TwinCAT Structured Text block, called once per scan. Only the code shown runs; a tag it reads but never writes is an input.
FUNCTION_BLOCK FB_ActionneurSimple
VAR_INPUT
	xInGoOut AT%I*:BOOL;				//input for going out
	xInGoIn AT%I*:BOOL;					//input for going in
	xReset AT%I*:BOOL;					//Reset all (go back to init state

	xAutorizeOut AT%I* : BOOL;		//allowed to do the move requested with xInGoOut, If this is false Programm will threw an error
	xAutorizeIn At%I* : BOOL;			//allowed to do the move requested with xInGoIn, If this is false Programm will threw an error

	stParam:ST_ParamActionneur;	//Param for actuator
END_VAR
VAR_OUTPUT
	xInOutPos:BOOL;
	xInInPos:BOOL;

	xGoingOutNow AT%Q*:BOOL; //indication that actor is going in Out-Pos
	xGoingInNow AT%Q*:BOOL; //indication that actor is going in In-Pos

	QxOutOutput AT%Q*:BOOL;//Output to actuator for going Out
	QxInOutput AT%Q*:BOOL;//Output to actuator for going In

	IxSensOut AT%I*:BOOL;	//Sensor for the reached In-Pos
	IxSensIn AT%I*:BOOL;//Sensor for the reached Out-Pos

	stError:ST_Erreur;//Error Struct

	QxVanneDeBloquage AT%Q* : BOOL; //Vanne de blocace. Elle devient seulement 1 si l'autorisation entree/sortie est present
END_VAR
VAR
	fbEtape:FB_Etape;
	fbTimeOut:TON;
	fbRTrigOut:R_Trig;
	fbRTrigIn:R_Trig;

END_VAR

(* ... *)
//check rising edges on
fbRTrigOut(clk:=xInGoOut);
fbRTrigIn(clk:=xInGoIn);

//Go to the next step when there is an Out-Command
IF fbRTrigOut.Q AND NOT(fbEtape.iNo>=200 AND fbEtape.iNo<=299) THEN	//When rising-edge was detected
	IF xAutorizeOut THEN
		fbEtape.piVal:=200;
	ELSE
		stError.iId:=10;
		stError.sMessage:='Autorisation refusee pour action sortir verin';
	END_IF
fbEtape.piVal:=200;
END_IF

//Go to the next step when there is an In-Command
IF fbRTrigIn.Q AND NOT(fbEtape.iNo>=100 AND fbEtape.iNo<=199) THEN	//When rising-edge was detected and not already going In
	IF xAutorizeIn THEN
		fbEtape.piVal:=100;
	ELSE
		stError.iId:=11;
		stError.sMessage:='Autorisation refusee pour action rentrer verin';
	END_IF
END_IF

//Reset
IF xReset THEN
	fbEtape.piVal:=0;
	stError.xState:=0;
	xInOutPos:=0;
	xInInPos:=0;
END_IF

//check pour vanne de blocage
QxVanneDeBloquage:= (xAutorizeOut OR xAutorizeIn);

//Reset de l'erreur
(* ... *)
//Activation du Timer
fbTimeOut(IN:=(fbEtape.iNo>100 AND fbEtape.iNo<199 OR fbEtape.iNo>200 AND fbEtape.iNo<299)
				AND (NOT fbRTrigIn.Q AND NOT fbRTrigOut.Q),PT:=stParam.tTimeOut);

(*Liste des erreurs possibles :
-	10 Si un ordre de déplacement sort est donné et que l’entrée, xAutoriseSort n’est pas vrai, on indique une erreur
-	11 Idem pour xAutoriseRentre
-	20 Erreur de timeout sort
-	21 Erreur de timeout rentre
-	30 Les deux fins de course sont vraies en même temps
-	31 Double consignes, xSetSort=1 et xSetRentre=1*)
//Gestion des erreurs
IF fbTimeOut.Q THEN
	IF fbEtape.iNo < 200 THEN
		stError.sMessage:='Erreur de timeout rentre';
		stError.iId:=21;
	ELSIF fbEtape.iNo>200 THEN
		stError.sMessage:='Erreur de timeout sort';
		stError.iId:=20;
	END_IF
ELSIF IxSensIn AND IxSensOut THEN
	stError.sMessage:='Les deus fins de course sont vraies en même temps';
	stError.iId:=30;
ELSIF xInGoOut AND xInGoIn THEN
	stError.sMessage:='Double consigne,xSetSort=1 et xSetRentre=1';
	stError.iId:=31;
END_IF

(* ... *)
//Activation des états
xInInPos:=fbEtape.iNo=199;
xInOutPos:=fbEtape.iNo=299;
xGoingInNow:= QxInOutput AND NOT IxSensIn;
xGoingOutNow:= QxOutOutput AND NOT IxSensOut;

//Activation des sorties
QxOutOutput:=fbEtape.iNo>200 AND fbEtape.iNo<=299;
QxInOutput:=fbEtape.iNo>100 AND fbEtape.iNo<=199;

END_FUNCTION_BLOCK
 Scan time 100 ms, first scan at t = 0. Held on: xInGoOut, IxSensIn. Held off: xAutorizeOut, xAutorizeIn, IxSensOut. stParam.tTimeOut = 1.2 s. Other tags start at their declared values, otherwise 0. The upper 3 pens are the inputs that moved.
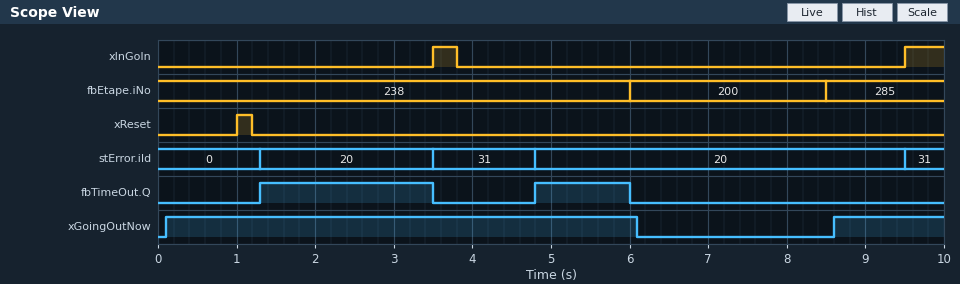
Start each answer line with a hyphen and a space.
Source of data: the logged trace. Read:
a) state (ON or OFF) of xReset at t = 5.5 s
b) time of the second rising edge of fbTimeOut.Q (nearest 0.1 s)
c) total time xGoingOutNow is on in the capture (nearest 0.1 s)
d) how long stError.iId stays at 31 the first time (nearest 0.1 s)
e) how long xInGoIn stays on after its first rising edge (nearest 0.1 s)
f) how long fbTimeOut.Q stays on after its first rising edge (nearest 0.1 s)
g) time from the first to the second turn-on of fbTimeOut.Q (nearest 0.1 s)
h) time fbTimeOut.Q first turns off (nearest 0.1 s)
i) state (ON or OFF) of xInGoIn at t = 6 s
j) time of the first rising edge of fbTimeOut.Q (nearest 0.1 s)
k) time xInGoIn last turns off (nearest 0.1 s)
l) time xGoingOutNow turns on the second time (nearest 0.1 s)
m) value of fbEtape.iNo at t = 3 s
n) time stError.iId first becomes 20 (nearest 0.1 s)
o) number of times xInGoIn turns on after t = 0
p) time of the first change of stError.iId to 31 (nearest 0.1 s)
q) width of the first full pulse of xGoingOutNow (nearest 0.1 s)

- OFF
- 4.8 s
- 7.4 s
- 1.3 s
- 0.3 s
- 2.2 s
- 3.5 s
- 3.5 s
- OFF
- 1.3 s
- 3.8 s
- 8.6 s
- 238
- 1.3 s
- 2
- 3.5 s
- 6.0 s
